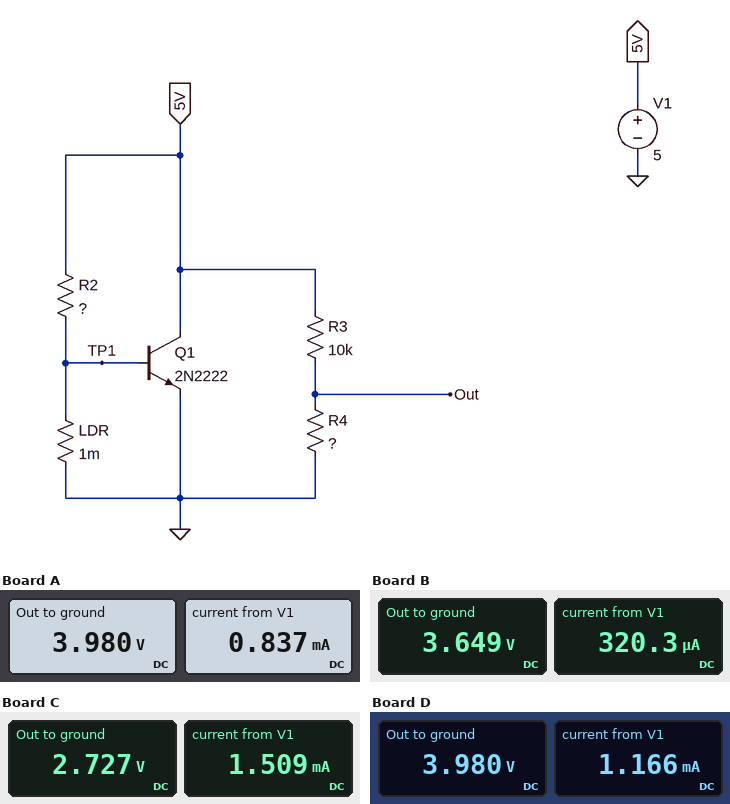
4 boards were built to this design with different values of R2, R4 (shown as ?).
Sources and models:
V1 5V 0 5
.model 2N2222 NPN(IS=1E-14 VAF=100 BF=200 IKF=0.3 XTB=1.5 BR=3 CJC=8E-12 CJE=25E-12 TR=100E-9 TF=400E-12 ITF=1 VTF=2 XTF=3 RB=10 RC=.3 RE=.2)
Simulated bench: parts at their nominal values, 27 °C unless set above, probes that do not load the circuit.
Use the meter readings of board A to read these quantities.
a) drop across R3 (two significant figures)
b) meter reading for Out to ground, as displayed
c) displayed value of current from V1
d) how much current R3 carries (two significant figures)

1.0 V
3.980 V
0.837 mA
100 µA
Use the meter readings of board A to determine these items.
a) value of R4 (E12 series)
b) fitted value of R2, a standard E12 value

39 kΩ
6.8 kΩ
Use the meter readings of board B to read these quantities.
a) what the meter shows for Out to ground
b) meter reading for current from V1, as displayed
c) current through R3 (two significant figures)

3.649 V
320.3 µA
140 µA
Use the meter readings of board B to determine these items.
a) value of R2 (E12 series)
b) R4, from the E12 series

27 kΩ
27 kΩ
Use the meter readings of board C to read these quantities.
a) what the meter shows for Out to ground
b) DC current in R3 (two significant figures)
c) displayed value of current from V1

2.727 V
230 µA
1.509 mA
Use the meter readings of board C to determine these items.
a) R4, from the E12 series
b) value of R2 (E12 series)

12 kΩ
3.9 kΩ
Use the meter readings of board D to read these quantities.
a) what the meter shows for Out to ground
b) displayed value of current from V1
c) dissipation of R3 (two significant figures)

3.980 V
1.166 mA
100 µW
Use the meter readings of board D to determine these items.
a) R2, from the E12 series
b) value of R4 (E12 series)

4.7 kΩ
39 kΩ
